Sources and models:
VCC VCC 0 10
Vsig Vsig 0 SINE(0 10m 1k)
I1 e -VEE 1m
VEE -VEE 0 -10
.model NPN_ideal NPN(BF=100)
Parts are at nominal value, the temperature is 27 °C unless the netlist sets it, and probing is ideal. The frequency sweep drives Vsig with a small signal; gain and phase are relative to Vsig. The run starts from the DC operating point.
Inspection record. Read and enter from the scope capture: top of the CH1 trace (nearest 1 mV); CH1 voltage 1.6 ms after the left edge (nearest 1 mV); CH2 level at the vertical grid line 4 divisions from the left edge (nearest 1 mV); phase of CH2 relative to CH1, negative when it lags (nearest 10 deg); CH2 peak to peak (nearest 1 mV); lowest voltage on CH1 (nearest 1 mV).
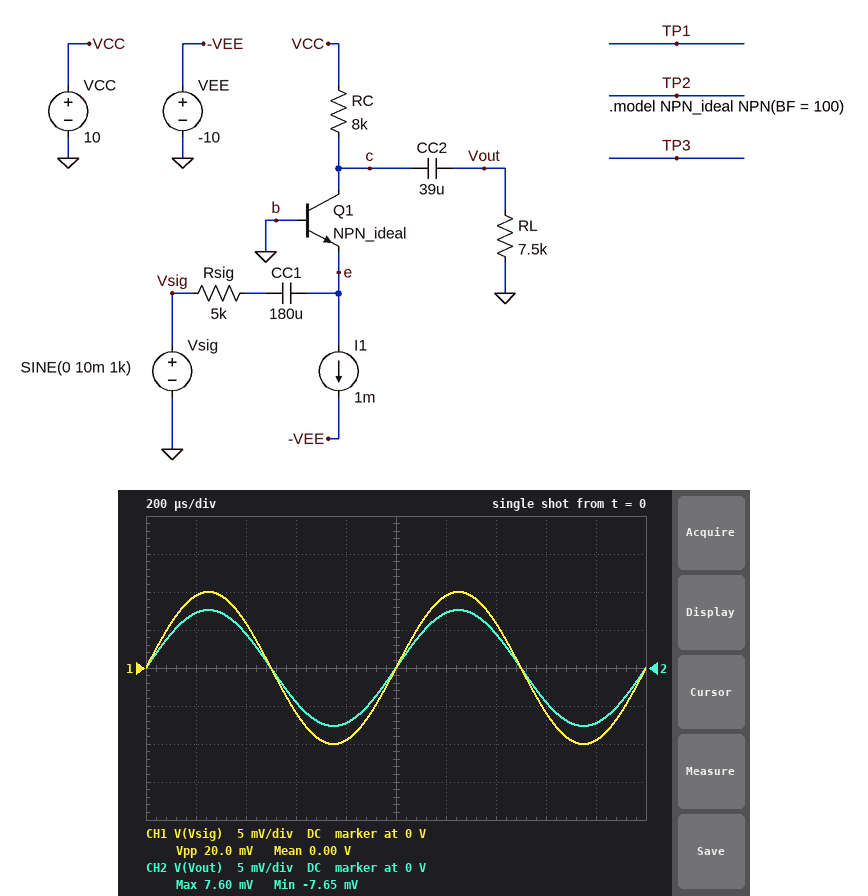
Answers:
10 mV
-6 mV
-7 mV
0 deg
15 mV
-10 mV
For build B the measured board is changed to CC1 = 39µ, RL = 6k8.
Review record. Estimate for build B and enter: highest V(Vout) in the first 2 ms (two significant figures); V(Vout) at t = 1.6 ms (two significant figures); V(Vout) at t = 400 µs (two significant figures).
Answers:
7.2 mV
-4.3 mV
4.2 mV
